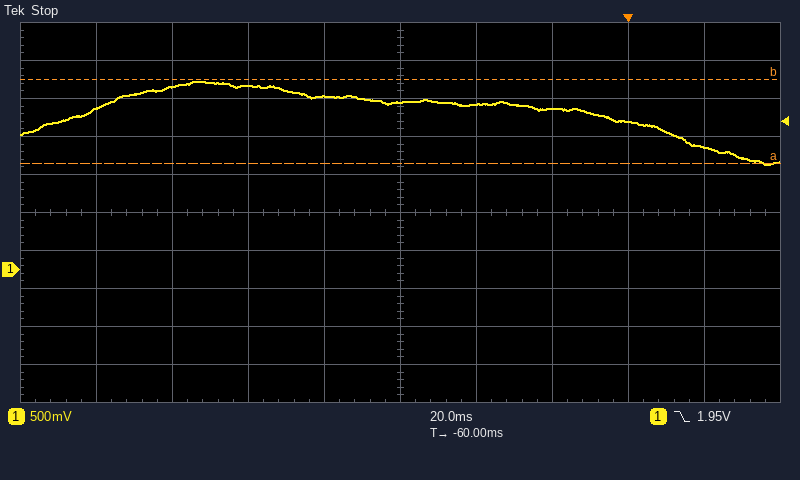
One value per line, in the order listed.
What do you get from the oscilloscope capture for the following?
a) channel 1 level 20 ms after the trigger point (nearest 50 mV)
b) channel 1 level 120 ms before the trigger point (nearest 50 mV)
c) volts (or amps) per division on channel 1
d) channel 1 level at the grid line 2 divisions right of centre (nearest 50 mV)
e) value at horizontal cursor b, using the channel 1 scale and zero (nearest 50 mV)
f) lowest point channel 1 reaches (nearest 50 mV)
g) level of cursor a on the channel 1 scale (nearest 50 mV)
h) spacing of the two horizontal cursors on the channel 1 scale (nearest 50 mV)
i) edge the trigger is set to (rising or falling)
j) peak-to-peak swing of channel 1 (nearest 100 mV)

1.60 V
2.40 V
500 mV
2.10 V
2.50 V
1.40 V
1.40 V
1.10 V
falling
1.10 V
